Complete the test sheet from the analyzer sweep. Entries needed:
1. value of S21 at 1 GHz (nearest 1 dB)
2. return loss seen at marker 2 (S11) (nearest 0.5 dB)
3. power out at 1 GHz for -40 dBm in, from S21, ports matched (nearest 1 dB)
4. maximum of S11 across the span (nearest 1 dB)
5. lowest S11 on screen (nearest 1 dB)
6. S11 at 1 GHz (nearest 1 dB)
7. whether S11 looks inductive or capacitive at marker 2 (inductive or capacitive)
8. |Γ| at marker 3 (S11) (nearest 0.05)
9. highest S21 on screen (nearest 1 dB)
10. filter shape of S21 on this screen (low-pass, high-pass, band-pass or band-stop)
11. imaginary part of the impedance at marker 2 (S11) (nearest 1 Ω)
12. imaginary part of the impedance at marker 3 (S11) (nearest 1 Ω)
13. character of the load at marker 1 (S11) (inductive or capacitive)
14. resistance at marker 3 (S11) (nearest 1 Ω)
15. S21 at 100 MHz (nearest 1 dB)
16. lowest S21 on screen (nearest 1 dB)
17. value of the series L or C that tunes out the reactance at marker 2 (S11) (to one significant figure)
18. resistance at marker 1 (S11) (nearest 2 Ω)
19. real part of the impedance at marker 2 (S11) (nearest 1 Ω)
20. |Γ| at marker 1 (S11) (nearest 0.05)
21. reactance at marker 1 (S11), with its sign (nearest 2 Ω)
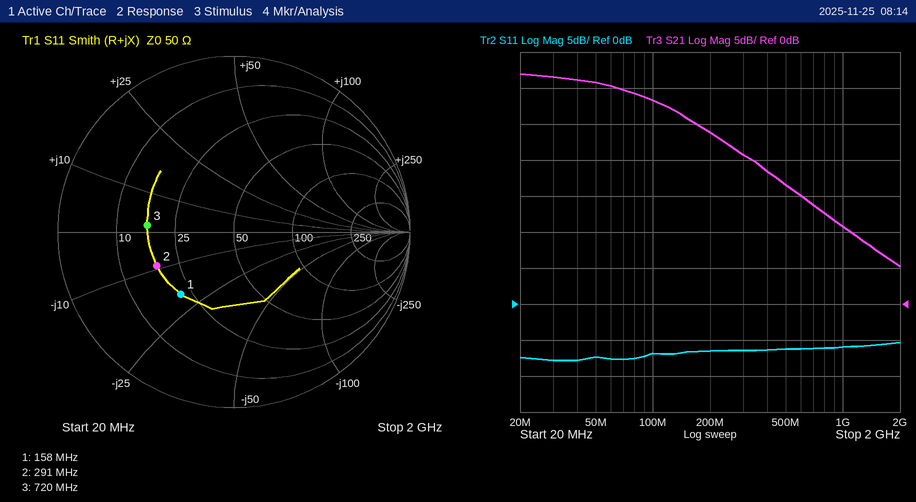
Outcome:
11 dB
6.5 dB
-29 dBm
-5 dB
-8 dB
-6 dB
capacitive
0.50
32 dB
low-pass
-9 Ω
+2 Ω
capacitive
17 Ω
28 dB
5 dB
5 nH
22 Ω
18 Ω
0.45
-20 Ω
